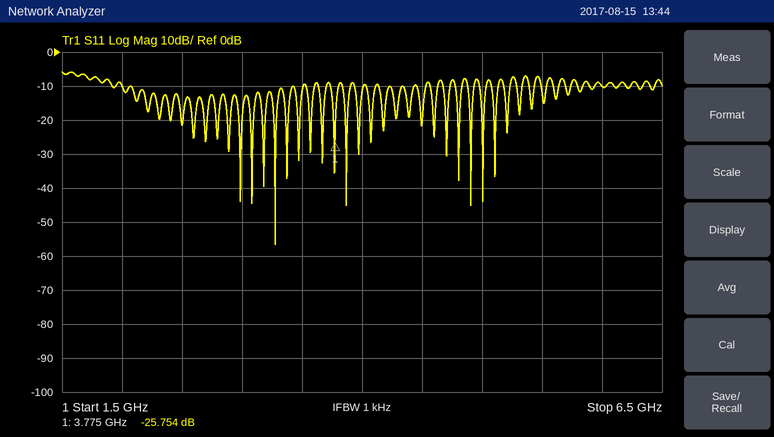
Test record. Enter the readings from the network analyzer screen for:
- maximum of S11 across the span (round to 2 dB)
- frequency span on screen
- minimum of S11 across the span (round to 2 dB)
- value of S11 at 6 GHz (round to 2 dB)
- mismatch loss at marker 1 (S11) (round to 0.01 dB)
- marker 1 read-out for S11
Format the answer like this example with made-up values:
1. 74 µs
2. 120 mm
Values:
1. -6 dB
2. 5 GHz
3. -56 dB
4. -10 dB
5. 0.01 dB
6. -25.754 dB
